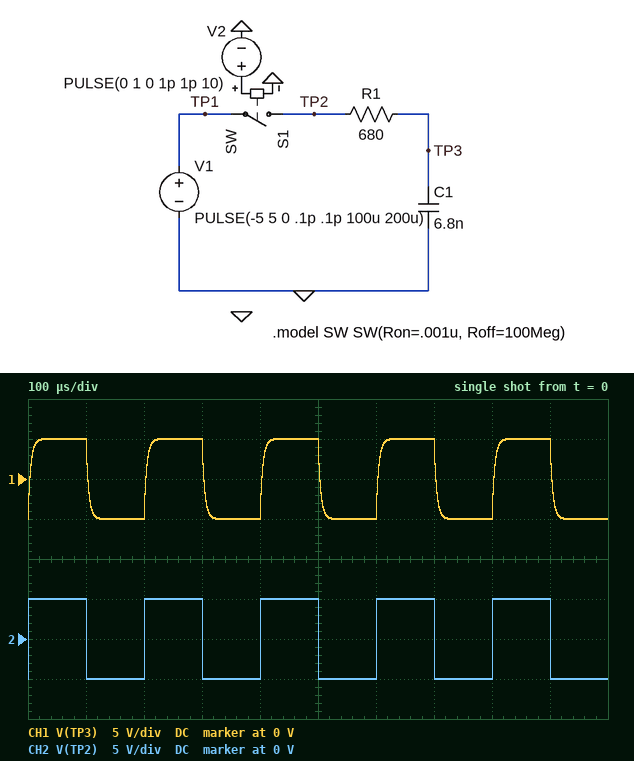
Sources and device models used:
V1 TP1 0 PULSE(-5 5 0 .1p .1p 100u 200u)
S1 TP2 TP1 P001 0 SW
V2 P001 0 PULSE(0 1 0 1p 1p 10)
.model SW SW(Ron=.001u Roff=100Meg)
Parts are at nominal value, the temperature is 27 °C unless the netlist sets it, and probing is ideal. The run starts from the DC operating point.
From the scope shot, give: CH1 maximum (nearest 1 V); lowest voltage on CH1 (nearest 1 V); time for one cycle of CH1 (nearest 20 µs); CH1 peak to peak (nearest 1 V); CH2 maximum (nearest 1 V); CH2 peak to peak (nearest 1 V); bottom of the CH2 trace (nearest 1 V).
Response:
5 V
-5 V
200 µs
10 V
5 V
10 V
-5 V
